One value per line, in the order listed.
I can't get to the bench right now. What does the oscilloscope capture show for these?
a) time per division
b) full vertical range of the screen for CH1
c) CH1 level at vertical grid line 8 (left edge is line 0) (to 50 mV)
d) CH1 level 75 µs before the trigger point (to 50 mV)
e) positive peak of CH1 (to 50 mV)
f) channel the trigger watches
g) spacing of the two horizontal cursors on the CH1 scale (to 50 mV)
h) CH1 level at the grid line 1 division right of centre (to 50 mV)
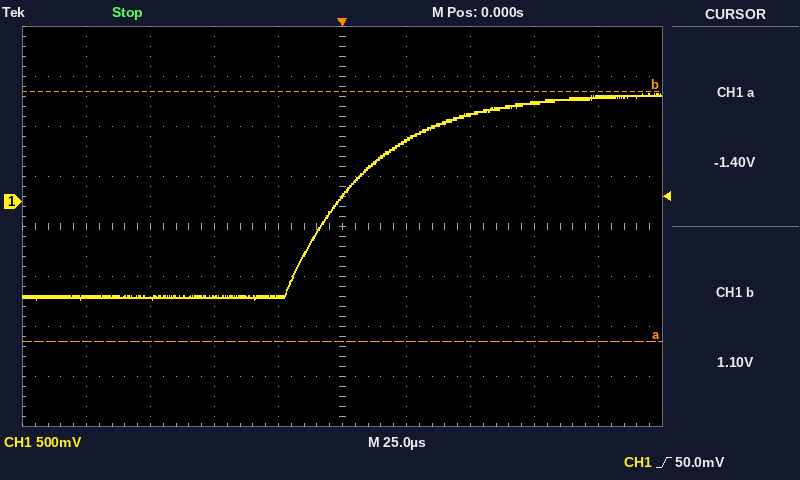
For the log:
25 µs
4 V
1.00 V
-950 mV
1.10 V
CH1
2.50 V
600 mV
